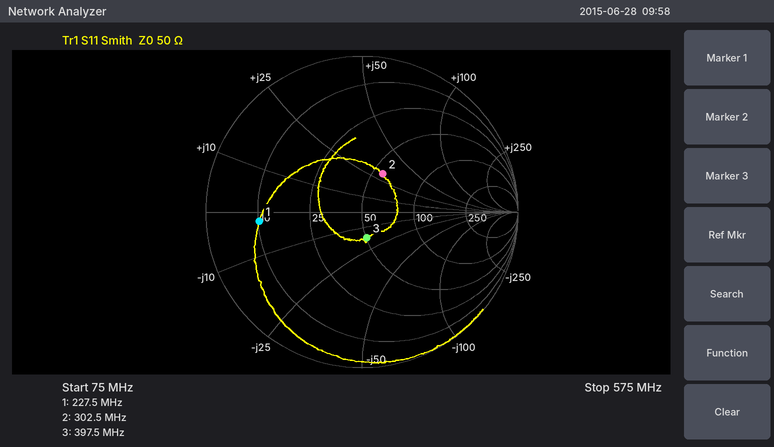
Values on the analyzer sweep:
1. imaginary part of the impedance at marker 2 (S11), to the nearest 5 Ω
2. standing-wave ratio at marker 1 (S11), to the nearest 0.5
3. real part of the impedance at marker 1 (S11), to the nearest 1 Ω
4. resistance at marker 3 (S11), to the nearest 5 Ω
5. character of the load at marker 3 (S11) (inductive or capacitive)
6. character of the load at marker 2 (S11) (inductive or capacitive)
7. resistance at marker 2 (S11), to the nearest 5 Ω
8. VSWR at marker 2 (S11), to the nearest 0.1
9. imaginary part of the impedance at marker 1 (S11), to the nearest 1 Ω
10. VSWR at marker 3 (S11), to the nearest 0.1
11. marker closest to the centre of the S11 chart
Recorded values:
+30 Ω
5.0
10 Ω
50 Ω
capacitive
inductive
55 Ω
1.8
-2 Ω
1.4
marker 3
